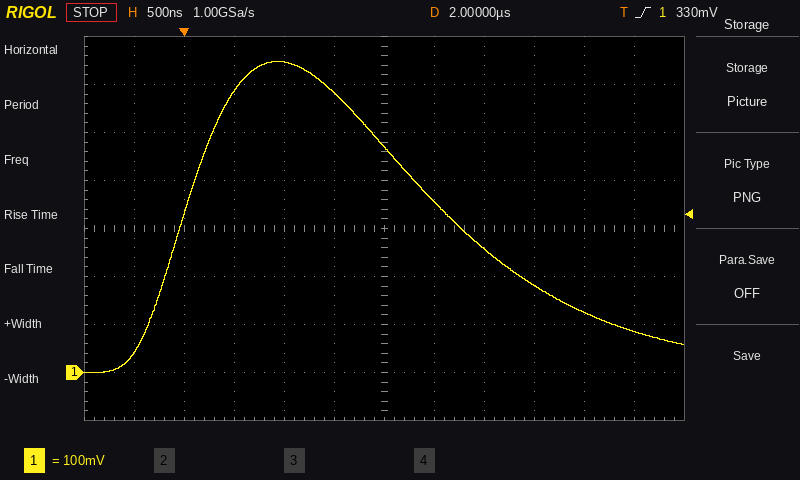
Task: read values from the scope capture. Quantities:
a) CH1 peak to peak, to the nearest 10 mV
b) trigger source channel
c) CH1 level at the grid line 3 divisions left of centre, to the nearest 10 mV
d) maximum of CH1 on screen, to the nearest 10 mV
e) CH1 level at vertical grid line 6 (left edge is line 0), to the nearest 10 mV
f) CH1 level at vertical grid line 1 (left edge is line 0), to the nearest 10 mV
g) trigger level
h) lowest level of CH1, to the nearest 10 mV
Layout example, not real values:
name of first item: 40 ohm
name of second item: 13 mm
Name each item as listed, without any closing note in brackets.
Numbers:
CH1 peak to peak, to the nearest 10 mV: 650 mV
trigger source channel: CH1
CH1 level at the grid line 3 divisions left of centre, to the nearest 10 mV: 590 mV
maximum of CH1 on screen, to the nearest 10 mV: 650 mV
CH1 level at vertical grid line 6 (left edge is line 0), to the nearest 10 mV: 470 mV
CH1 level at vertical grid line 1 (left edge is line 0), to the nearest 10 mV: 40 mV
trigger level: 330 mV
lowest level of CH1, to the nearest 10 mV: 0 mV
